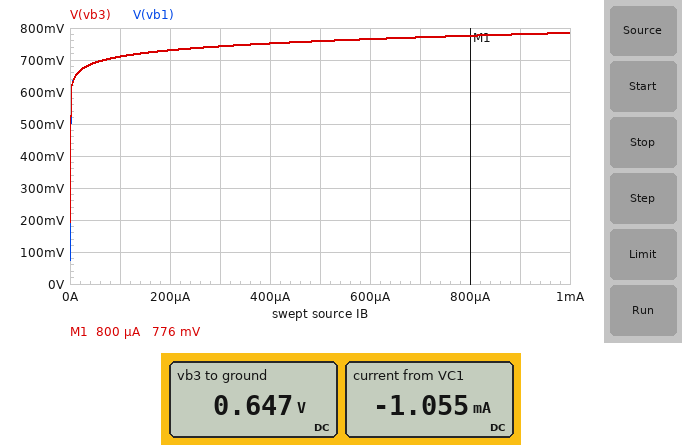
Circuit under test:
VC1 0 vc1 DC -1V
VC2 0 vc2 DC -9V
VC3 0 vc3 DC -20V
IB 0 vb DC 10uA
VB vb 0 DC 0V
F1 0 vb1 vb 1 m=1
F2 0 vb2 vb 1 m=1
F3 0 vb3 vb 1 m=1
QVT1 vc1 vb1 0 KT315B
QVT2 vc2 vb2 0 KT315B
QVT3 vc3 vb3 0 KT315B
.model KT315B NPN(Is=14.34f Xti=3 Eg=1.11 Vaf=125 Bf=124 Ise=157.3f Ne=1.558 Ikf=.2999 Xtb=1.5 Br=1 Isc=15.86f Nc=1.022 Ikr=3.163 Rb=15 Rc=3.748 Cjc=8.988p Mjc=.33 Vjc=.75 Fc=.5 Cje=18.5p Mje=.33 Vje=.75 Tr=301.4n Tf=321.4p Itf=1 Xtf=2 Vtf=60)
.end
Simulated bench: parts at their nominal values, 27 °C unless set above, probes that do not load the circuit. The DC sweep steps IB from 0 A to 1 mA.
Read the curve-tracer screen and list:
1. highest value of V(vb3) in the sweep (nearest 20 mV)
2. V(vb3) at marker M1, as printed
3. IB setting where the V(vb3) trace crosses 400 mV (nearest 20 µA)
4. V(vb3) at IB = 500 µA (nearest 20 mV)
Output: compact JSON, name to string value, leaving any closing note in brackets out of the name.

{"highest value of V(vb3) in the sweep": "780 mV", "V(vb3) at marker M1, as printed": "776 mV", "IB setting where the V(vb3) trace crosses 400 mV": "0 A", "V(vb3) at IB = 500 µA": "760 mV"}
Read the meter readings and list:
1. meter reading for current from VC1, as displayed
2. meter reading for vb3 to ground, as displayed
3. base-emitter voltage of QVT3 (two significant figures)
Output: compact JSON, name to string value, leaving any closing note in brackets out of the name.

{"meter reading for current from VC1, as displayed": "-1.055 mA", "meter reading for vb3 to ground, as displayed": "0.647 V", "base-emitter voltage of QVT3": "650 mV"}
